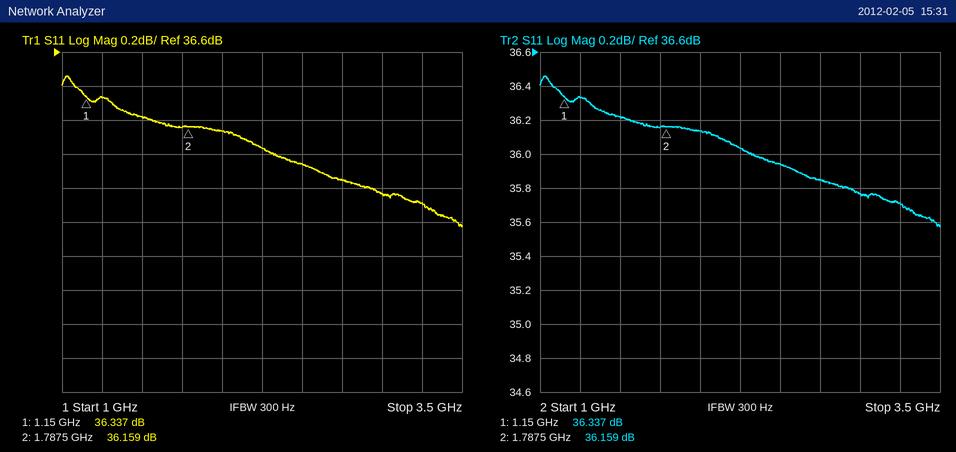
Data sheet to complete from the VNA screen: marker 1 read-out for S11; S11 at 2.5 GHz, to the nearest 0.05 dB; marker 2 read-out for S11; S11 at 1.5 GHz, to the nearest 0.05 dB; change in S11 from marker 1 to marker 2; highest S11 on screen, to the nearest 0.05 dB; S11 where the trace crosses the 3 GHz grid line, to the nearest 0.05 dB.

36.337 dB
35.95 dB
36.159 dB
36.20 dB
-0.178 dB
36.45 dB
35.75 dB
